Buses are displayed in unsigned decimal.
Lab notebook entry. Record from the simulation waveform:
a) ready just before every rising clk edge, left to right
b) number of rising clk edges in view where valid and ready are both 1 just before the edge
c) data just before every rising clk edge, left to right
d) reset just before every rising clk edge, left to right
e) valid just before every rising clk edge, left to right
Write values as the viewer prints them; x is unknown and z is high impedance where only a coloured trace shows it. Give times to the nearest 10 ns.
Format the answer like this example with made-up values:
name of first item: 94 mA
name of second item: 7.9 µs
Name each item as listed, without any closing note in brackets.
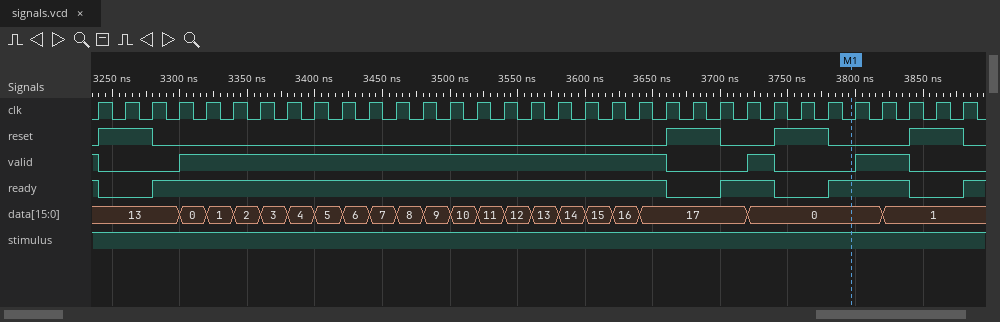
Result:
ready just before every rising clk edge, left to right: 1 0 0 1 1 1 1 1 1 1 1 1 1 1 1 1 1 1 1 1 1 1 0 0 1 1 0 0 1 1 1 0 0
number of rising clk edges in view where valid and ready are both 1 just before the edge: 22
data just before every rising clk edge, left to right: 13, 13, 13, 13, 0, 1, 2, 3, 4, 5, 6, 7, 8, 9, 10, 11, 12, 13, 14, 15, 16, 17, 17, 17, 17, 0, 0, 0, 0, 0, 1, 1, 1
reset just before every rising clk edge, left to right: 0 1 1 0 0 0 0 0 0 0 0 0 0 0 0 0 0 0 0 0 0 0 1 1 0 0 1 1 0 0 0 1 1
valid just before every rising clk edge, left to right: 1 0 0 0 1 1 1 1 1 1 1 1 1 1 1 1 1 1 1 1 1 1 0 0 0 1 0 0 0 1 1 0 0
